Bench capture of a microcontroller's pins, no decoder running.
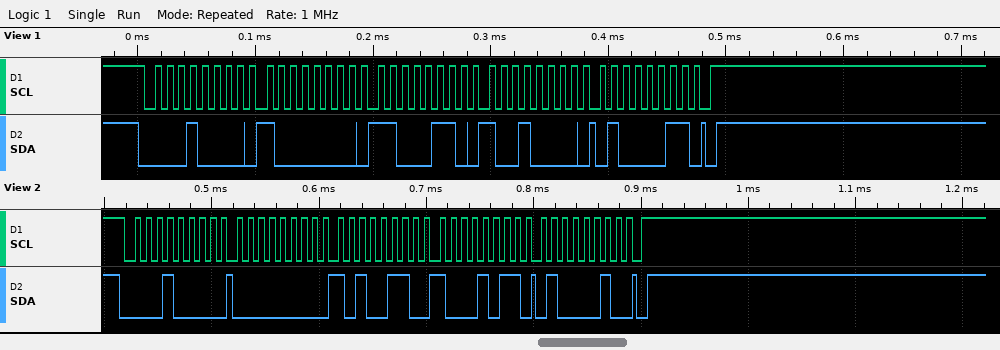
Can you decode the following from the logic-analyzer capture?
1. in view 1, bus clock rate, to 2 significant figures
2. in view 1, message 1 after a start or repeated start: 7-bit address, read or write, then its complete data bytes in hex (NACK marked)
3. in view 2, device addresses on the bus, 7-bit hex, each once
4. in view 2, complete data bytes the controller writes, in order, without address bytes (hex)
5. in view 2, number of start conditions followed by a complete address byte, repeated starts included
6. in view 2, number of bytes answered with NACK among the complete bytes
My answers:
100 kHz
0x08 write: 80 C6 90 43
0x08
00 A6 8B 42
1
0
